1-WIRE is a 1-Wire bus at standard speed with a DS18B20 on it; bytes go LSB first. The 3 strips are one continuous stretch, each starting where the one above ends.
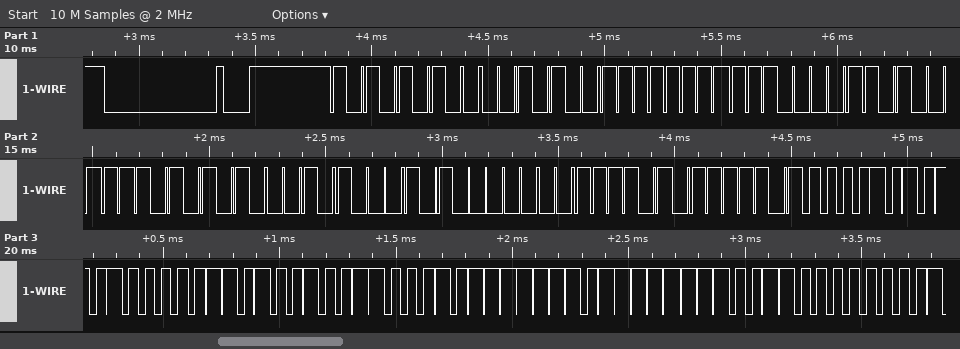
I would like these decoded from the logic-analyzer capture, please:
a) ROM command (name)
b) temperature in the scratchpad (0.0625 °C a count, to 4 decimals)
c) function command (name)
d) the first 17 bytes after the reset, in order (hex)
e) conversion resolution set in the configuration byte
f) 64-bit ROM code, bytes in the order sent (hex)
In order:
Match ROM
85.0000 °C
Read Scratchpad
55 28 FF 87 E5 55 14 05 BC BE 50 05 4B 46 7F FF 0C
12 bits
28 FF 87 E5 55 14 05 BC
